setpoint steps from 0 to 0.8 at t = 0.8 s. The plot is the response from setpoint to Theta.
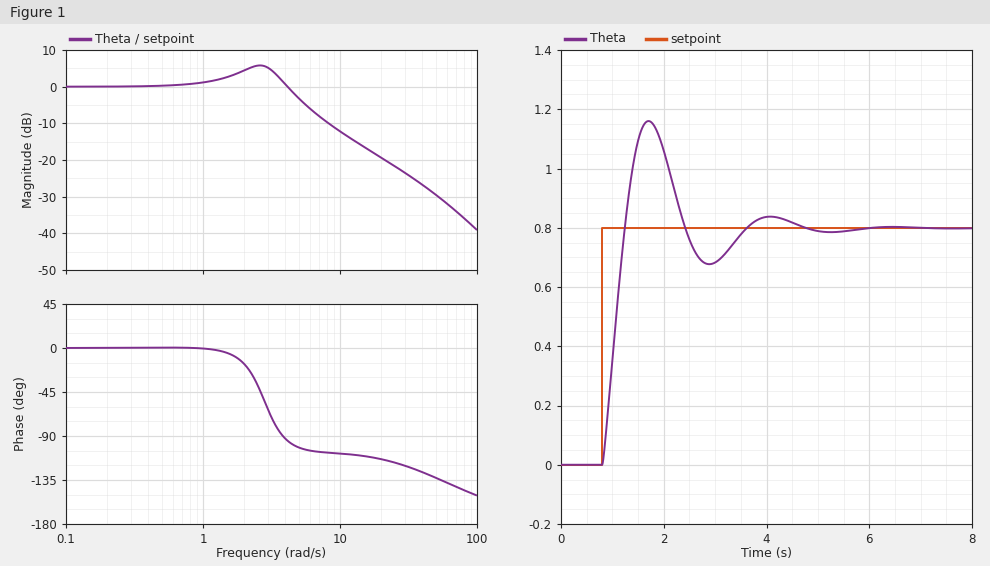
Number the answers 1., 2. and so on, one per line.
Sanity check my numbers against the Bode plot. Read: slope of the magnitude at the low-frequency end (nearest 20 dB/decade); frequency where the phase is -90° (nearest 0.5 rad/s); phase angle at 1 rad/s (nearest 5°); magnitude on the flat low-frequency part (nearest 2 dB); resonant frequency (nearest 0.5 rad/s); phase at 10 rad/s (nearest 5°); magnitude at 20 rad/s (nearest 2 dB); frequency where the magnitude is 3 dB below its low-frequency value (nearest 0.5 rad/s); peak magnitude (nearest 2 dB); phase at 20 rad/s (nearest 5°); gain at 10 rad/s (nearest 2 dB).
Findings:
1. 0 dB/decade
2. 4.0 rad/s
3. 0°
4. 0 dB
5. 2.5 rad/s
6. -110°
7. -20 dB
8. 5.0 rad/s
9. 6 dB
10. -115°
11. -12 dB
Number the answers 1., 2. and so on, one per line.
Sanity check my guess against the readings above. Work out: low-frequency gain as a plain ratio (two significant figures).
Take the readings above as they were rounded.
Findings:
1. 1.0
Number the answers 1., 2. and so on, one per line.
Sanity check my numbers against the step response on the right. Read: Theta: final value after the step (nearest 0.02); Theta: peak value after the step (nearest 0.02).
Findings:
1. 0.80
2. 1.16
